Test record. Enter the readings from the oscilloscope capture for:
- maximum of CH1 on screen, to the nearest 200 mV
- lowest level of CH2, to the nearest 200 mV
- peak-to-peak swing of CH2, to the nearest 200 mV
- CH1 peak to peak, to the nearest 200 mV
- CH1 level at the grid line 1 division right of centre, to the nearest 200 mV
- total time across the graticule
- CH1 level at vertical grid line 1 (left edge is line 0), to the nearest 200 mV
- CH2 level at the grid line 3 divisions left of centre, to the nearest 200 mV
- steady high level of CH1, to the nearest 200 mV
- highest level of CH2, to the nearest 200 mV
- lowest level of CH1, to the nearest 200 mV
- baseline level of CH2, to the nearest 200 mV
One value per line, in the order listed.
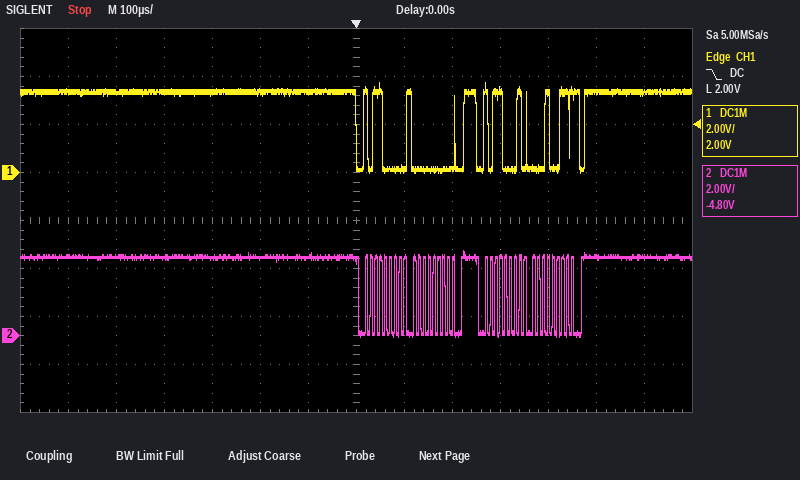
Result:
3.8 V
0.0 V
3.6 V
3.8 V
200 mV
1.4 ms
3.4 V
3.2 V
3.4 V
3.6 V
0.0 V
3.2 V
